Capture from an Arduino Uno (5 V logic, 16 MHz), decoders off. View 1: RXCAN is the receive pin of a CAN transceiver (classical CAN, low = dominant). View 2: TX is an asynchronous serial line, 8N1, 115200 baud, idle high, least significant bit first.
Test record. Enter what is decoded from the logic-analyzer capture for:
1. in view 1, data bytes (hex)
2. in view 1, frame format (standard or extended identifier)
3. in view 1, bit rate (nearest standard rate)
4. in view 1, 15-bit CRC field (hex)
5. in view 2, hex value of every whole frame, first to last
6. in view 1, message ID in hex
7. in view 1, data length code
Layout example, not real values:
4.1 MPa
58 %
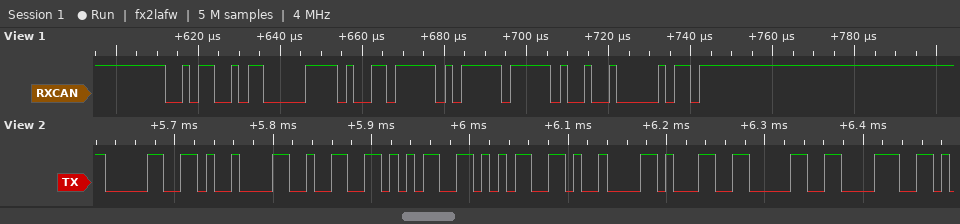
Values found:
A6 FD FF
standard
500 kbit/s
0x6481
30 09 32 35 35 09 31 30 38
0x2CB
3
